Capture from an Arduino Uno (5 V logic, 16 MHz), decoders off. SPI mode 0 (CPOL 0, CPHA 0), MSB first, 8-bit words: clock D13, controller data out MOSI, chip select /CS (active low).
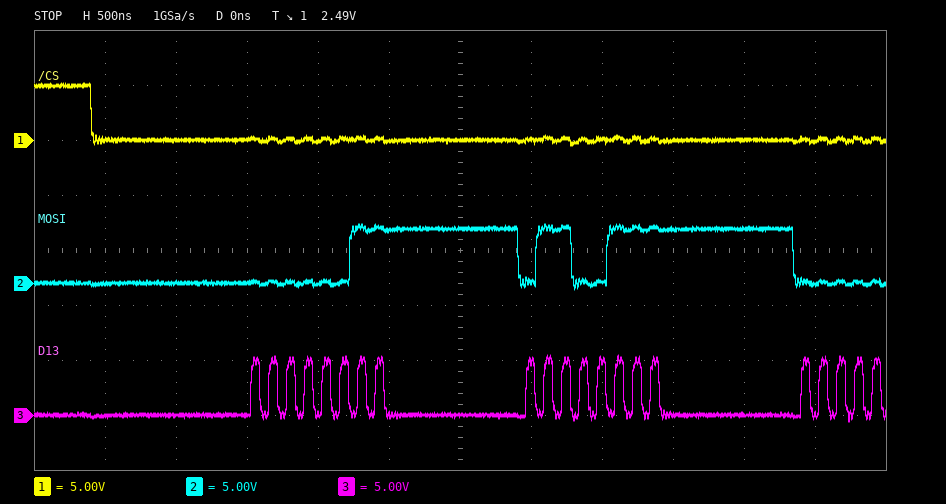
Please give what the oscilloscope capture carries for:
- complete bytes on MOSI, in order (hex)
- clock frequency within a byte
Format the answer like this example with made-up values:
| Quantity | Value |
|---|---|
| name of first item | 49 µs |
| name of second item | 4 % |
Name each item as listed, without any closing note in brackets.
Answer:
| Quantity | Value |
|---|---|
| complete bytes on MOSI, in order | 03 67 |
| clock frequency within a byte | 8 MHz |
